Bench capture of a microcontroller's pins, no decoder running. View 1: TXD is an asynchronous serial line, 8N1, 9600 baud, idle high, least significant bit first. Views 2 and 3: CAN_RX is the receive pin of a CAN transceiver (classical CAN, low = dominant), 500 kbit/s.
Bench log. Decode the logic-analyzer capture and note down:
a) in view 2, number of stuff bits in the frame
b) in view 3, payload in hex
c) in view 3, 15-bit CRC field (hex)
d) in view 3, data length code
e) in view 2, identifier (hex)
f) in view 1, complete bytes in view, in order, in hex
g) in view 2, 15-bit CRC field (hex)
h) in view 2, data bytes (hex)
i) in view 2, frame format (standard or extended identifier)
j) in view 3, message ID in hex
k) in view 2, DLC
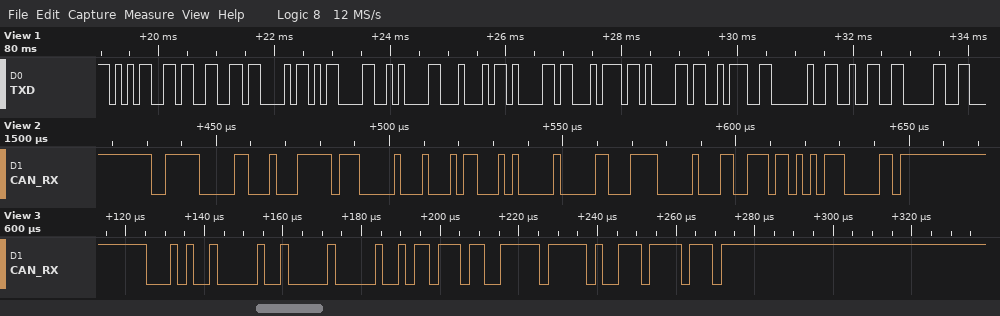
8
00 2D D9 FF
0x677B
4
0x3E1
35 33 43 0D 0A 44 61 74 61 3A 20 32 30
0x6AE0
FF 00 8B 14 00 8F 00 CE
standard
0x148
8
